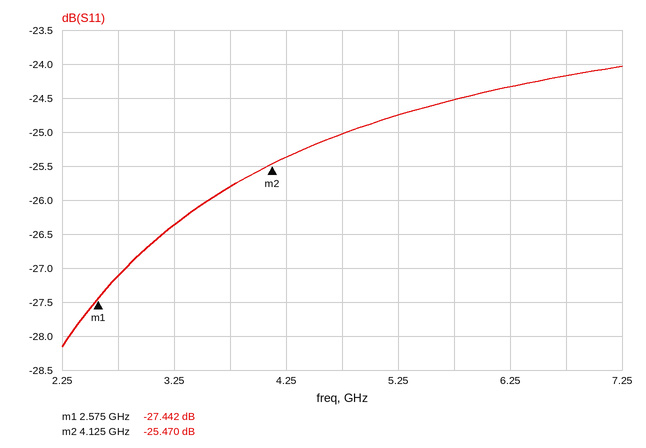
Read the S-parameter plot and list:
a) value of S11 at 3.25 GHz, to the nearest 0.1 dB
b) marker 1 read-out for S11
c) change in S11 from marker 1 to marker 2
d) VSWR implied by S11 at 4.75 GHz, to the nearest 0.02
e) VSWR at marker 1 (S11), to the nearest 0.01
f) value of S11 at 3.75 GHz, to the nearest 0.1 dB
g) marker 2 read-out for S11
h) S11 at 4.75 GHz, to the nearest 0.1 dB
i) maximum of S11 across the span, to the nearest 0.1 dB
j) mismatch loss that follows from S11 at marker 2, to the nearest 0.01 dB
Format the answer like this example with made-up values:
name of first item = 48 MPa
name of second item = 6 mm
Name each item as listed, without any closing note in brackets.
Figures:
value of S11 at 3.25 GHz, to the nearest 0.1 dB = -26.4 dB
marker 1 read-out for S11 = -27.442 dB
change in S11 from marker 1 to marker 2 = 1.972 dB
VSWR implied by S11 at 4.75 GHz, to the nearest 0.02 = 1.12
VSWR at marker 1 (S11), to the nearest 0.01 = 1.09
value of S11 at 3.75 GHz, to the nearest 0.1 dB = -25.8 dB
marker 2 read-out for S11 = -25.470 dB
S11 at 4.75 GHz, to the nearest 0.1 dB = -25.0 dB
maximum of S11 across the span, to the nearest 0.1 dB = -24.0 dB
mismatch loss that follows from S11 at marker 2, to the nearest 0.01 dB = 0.01 dB
